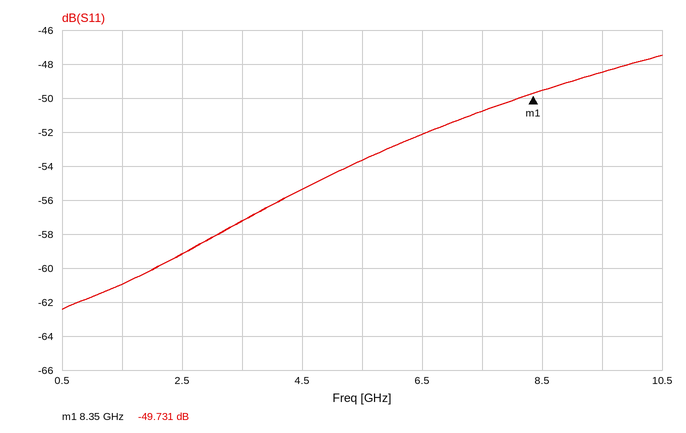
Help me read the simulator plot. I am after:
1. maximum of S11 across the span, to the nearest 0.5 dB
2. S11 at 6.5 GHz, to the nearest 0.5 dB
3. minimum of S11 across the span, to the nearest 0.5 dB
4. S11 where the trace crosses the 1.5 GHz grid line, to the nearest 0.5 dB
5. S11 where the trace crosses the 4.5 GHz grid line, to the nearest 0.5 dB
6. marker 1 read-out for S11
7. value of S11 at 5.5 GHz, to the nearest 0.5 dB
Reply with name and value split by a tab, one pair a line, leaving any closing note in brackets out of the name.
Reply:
maximum of S11 across the span, to the nearest 0.5 dB	-47.5 dB
S11 at 6.5 GHz, to the nearest 0.5 dB	-52.0 dB
minimum of S11 across the span, to the nearest 0.5 dB	-62.5 dB
S11 where the trace crosses the 1.5 GHz grid line, to the nearest 0.5 dB	-61.0 dB
S11 where the trace crosses the 4.5 GHz grid line, to the nearest 0.5 dB	-55.5 dB
marker 1 read-out for S11	-49.731 dB
value of S11 at 5.5 GHz, to the nearest 0.5 dB	-53.5 dB
